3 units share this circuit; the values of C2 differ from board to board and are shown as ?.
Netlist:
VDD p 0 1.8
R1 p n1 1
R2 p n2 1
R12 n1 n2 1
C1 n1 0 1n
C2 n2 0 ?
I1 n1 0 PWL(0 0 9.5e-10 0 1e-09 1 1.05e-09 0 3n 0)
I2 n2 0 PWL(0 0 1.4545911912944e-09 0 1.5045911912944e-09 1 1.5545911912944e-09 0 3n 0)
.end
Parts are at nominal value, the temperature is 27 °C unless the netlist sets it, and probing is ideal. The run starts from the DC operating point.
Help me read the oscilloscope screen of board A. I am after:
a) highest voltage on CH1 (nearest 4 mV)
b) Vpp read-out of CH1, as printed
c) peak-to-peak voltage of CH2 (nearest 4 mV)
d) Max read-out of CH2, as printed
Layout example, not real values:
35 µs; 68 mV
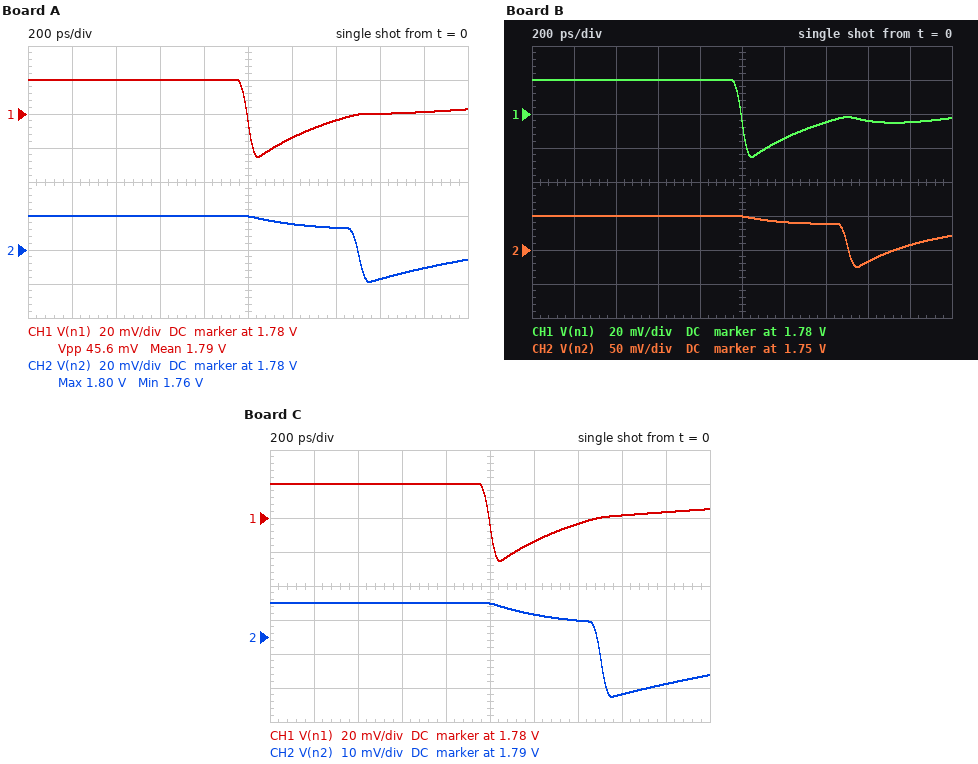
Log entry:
1.800 V; 45.6 mV; 40 mV; 1.80 V
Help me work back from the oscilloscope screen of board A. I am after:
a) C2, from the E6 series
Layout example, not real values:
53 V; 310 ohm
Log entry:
1.5 nF
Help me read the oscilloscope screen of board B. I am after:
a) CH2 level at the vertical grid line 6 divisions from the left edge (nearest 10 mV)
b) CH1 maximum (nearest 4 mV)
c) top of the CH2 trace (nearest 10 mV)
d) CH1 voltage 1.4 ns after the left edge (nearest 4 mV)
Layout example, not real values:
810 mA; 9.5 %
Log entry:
1.79 V; 1.800 V; 1.80 V; 1.776 V
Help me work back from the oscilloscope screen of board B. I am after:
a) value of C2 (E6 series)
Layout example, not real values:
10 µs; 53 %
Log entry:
680 pF
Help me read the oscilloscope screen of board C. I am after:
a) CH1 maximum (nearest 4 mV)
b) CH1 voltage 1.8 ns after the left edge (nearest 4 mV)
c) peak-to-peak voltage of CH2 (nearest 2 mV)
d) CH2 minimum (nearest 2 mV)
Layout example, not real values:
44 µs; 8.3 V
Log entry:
1.800 V; 1.784 V; 28 mV; 1.772 V
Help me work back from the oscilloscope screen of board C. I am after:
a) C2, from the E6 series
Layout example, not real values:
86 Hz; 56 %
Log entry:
2.2 nF
